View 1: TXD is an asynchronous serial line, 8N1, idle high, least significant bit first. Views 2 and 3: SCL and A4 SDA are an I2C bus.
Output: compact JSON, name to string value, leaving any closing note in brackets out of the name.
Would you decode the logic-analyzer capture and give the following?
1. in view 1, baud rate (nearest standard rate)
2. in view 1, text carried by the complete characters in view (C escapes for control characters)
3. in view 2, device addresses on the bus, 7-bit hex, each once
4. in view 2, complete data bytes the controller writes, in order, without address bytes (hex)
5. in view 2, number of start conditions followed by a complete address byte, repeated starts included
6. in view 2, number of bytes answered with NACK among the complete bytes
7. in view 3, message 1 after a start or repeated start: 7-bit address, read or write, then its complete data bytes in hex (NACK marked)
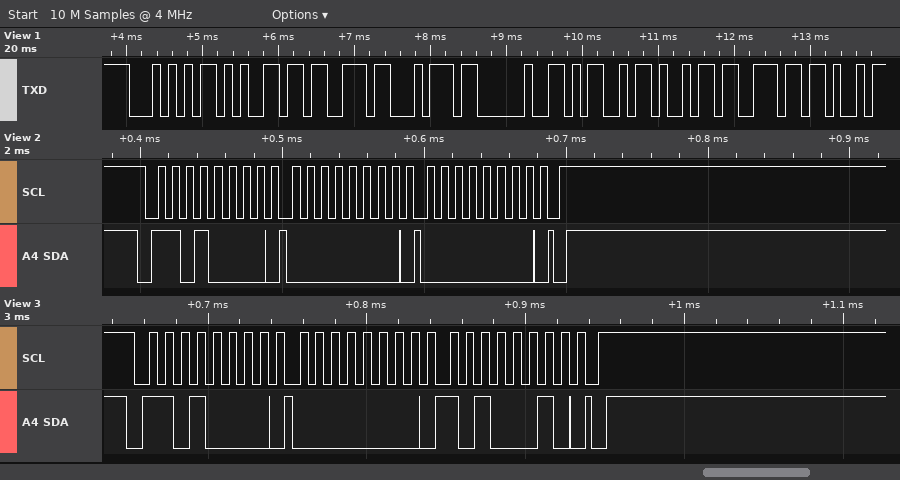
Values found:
{"in view 1, baud rate": "9600 baud", "in view 1, text carried by the complete characters in view": "\"Test Min\"", "in view 2, device addresses on the bus, 7-bit hex, each once": "0x68", "in view 2, complete data bytes the controller writes, in order, without address bytes": "00 00", "in view 2, number of start conditions followed by a complete address byte, repeated starts included": "1", "in view 2, number of bytes answered with NACK among the complete bytes": "0", "in view 3, message 1 after a start or repeated start: 7-bit address, read or write, then its complete data bytes in hex": "0x68 write: 00 A2"}
